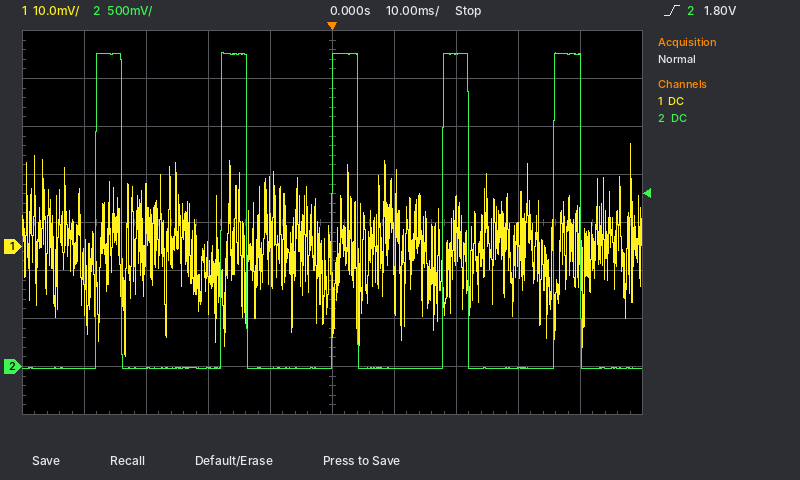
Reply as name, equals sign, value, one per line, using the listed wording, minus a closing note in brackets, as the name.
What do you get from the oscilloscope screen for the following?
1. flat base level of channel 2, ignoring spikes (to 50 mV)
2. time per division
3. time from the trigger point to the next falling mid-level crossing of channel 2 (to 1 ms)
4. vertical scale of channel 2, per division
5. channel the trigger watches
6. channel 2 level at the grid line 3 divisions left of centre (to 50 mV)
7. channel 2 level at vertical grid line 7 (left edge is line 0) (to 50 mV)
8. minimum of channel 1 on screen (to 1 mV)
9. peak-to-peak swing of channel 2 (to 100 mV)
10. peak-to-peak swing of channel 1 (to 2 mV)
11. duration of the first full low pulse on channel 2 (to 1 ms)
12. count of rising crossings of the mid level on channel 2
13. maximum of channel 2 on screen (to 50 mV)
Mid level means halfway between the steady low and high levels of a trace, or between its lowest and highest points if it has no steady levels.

flat base level of channel 2, ignoring spikes = 0 mV
time per division = 10 ms
time from the trigger point to the next falling mid-level crossing of channel 2 = 4 ms
vertical scale of channel 2, per division = 500 mV
channel the trigger watches = channel 2
channel 2 level at the grid line 3 divisions left of centre = 0 mV
channel 2 level at vertical grid line 7 (left edge is line 0) = 3.25 V
minimum of channel 1 on screen = -23 mV
peak-to-peak swing of channel 2 = 3.30 V
peak-to-peak swing of channel 1 = 44 mV
duration of the first full low pulse on channel 2 = 16 ms
count of rising crossings of the mid level on channel 2 = 5
maximum of channel 2 on screen = 3.25 V
